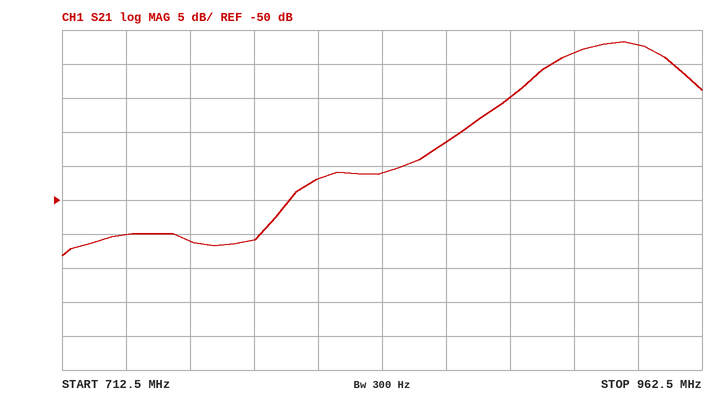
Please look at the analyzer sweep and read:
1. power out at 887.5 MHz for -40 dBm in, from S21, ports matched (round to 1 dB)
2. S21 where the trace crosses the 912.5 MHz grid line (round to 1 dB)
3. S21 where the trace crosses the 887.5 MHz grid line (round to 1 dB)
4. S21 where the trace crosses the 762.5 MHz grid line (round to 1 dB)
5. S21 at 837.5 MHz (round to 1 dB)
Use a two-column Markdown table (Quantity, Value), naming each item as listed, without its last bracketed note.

| Quantity | Value |
|---|---|
| power out at 887.5 MHz for -40 dBm in, from S21, ports matched | -75 dBm |
| S21 where the trace crosses the 912.5 MHz grid line | -28 dB |
| S21 where the trace crosses the 887.5 MHz grid line | -35 dB |
| S21 where the trace crosses the 762.5 MHz grid line | -56 dB |
| S21 at 837.5 MHz | -46 dB |
